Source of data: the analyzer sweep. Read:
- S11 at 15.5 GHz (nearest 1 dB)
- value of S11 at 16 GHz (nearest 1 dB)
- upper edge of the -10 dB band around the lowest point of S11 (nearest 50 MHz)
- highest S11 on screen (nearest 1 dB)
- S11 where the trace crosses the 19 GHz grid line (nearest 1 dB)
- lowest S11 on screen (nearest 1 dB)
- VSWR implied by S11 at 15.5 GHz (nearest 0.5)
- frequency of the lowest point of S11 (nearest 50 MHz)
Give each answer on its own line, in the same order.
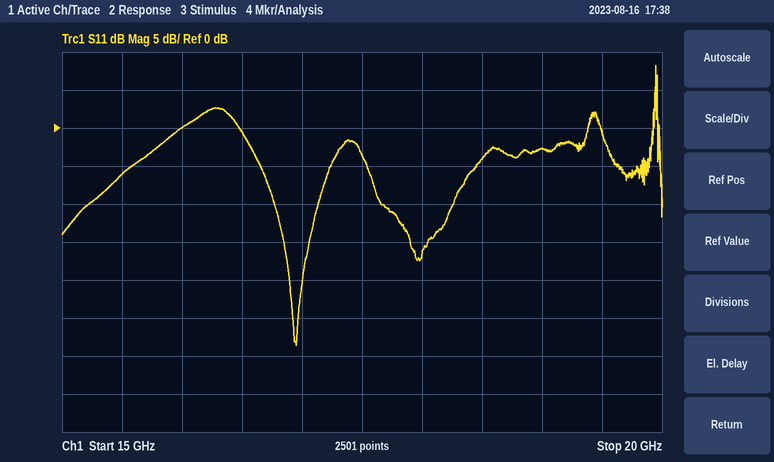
-6 dB
0 dB
17.15 GHz
8 dB
-3 dB
-29 dB
3.0
16.95 GHz
